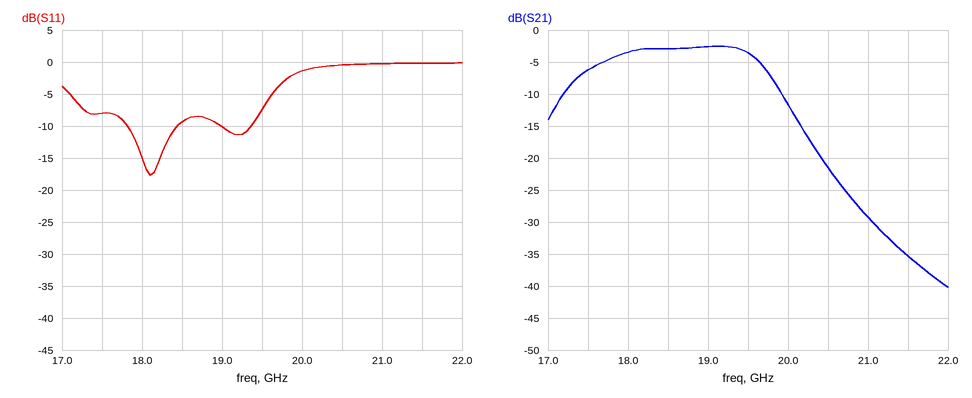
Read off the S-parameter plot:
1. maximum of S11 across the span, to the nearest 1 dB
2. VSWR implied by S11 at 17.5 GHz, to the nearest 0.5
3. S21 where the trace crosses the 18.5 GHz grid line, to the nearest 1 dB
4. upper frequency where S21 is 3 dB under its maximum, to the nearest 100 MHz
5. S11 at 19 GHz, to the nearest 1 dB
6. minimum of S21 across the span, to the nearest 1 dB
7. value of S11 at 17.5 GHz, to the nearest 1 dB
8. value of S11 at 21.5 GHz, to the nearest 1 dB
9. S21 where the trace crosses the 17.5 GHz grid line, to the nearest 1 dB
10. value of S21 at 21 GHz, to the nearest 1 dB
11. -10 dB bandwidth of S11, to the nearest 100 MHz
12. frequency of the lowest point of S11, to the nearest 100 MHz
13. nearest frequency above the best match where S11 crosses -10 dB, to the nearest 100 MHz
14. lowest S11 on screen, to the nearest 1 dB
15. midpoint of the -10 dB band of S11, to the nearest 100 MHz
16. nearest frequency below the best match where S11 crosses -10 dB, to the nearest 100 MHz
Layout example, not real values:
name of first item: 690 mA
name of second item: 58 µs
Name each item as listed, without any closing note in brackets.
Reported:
maximum of S11 across the span, to the nearest 1 dB: 0 dB
VSWR implied by S11 at 17.5 GHz, to the nearest 0.5: 2.5
S21 where the trace crosses the 18.5 GHz grid line, to the nearest 1 dB: -3 dB
upper frequency where S21 is 3 dB under its maximum, to the nearest 100 MHz: 19.7 GHz
S11 at 19 GHz, to the nearest 1 dB: -10 dB
minimum of S21 across the span, to the nearest 1 dB: -40 dB
value of S11 at 17.5 GHz, to the nearest 1 dB: -8 dB
value of S11 at 21.5 GHz, to the nearest 1 dB: 0 dB
S21 where the trace crosses the 17.5 GHz grid line, to the nearest 1 dB: -6 dB
value of S21 at 21 GHz, to the nearest 1 dB: -29 dB
-10 dB bandwidth of S11, to the nearest 100 MHz: 600 MHz
frequency of the lowest point of S11, to the nearest 100 MHz: 18.1 GHz
nearest frequency above the best match where S11 crosses -10 dB, to the nearest 100 MHz: 18.4 GHz
lowest S11 on screen, to the nearest 1 dB: -18 dB
midpoint of the -10 dB band of S11, to the nearest 100 MHz: 18.1 GHz
nearest frequency below the best match where S11 crosses -10 dB, to the nearest 100 MHz: 17.8 GHz
